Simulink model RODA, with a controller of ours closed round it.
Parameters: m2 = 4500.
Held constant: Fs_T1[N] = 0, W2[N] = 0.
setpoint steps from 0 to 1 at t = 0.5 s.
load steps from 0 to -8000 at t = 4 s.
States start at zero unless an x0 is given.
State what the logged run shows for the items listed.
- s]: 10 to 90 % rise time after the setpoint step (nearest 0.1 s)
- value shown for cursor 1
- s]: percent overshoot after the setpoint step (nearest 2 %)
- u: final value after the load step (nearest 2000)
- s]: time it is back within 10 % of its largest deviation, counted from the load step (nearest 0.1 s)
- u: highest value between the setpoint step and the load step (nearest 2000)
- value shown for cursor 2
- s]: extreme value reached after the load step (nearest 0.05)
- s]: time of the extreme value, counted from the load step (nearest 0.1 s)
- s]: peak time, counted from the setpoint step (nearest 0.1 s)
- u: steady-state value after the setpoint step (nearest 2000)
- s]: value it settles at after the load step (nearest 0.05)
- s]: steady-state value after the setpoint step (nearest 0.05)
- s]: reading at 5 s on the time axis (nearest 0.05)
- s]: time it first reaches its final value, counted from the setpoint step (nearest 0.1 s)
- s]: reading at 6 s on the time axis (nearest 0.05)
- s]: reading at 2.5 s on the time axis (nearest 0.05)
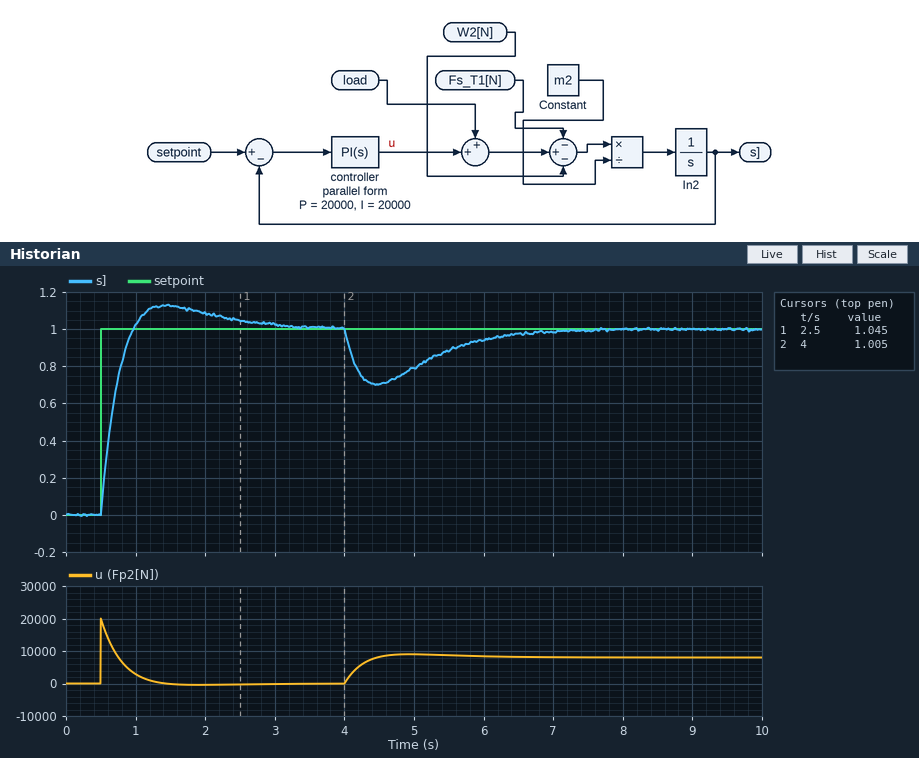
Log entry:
0.3 s
1.045
12 %
8000
2.4 s
20000
1.005
0.70
0.5 s
0.9 s
0
1.00
1.00
0.80
0.5 s
0.95
1.05
